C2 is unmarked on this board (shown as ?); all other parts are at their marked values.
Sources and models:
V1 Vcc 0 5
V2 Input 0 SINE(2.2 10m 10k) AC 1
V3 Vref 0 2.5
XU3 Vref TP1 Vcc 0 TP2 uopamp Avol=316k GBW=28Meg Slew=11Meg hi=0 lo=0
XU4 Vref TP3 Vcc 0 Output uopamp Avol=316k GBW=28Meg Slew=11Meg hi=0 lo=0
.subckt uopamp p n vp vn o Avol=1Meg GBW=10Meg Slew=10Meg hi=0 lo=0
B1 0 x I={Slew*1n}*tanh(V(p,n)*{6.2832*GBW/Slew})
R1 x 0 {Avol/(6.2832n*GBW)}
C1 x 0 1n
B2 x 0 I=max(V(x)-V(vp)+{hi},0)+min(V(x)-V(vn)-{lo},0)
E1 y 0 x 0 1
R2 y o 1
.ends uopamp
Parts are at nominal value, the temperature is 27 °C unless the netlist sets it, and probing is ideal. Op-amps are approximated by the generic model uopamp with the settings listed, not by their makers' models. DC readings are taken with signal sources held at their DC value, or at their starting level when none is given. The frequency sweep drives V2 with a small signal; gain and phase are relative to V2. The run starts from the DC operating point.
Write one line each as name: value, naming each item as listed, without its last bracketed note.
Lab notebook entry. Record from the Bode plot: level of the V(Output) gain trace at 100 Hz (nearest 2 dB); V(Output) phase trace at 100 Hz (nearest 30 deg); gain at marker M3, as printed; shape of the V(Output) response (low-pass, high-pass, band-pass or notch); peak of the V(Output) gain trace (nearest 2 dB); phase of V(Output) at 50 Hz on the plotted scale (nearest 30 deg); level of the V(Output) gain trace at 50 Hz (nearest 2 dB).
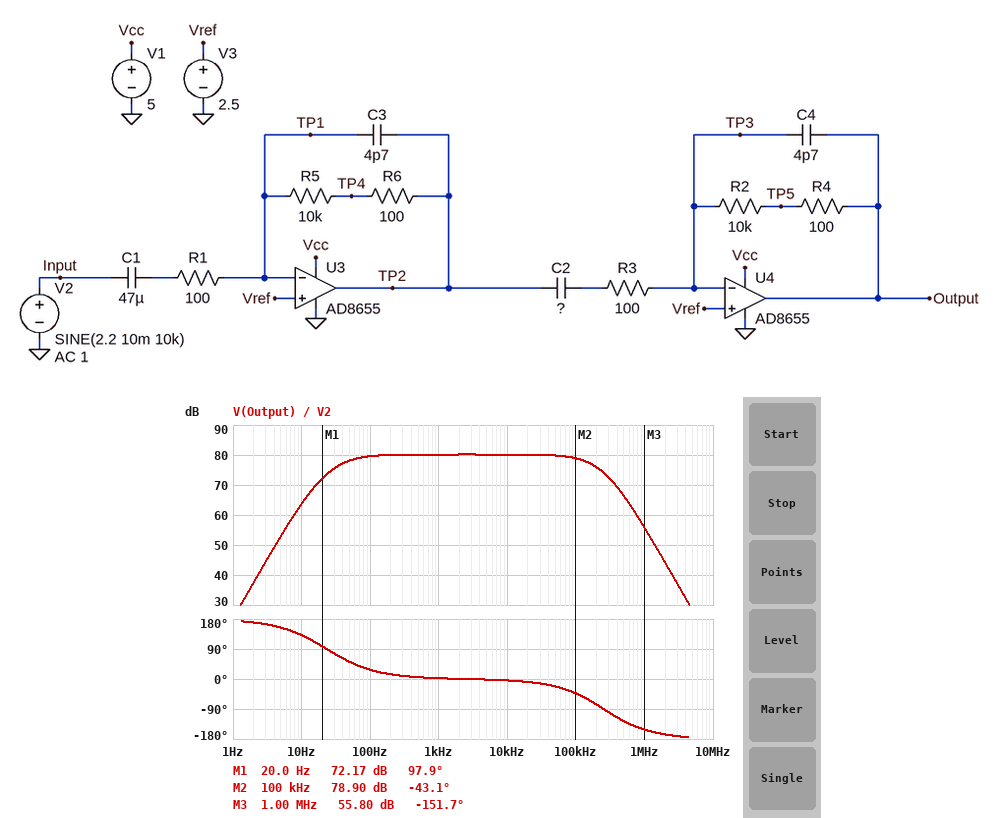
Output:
level of the V(Output) gain trace at 100 Hz: 80 dB
V(Output) phase trace at 100 Hz: 30 deg
gain at marker M3, as printed: 55.80 dB
shape of the V(Output) response: band-pass
peak of the V(Output) gain trace: 80 dB
phase of V(Output) at 50 Hz on the plotted scale: 60 deg
level of the V(Output) gain trace at 50 Hz: 78 dB
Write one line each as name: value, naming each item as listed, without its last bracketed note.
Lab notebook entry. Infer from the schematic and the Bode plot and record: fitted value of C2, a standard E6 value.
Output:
fitted value of C2, a standard E6 value: 100 µF
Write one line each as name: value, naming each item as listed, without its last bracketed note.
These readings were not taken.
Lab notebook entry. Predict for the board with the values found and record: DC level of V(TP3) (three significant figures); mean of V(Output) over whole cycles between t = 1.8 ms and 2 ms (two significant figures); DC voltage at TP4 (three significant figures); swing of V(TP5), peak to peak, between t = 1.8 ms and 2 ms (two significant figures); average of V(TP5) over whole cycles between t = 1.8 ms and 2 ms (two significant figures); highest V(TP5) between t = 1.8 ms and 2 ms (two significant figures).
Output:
DC level of V(TP3): 2.50 V
mean of V(Output) over whole cycles between t = 1.8 ms and 2 ms: 2.5 V
DC voltage at TP4: 2.50 V
swing of V(TP5), peak to peak, between t = 1.8 ms and 2 ms: 5.0 V
average of V(TP5) over whole cycles between t = 1.8 ms and 2 ms: 2.5 V
highest V(TP5) between t = 1.8 ms and 2 ms: 5.0 V
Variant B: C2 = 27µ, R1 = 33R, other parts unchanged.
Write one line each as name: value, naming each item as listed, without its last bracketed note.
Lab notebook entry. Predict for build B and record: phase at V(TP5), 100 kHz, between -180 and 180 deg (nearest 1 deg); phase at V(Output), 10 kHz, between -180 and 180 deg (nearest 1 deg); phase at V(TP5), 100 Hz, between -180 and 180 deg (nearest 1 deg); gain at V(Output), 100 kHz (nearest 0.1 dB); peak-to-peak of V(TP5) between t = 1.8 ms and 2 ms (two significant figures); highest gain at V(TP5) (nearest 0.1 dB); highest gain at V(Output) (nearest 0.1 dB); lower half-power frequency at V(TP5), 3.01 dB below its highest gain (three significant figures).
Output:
phase at V(TP5), 100 kHz, between -180 and 180 deg: -70 deg
phase at V(Output), 10 kHz, between -180 and 180 deg: -8 deg
phase at V(TP5), 100 Hz, between -180 and 180 deg: 76 deg
gain at V(Output), 100 kHz: 85.6 dB
peak-to-peak of V(TP5) between t = 1.8 ms and 2 ms: 5.0 V
highest gain at V(TP5): 89.7 dB
highest gain at V(Output): 89.8 dB
lower half-power frequency at V(TP5), 3.01 dB below its highest gain: 127 Hz
